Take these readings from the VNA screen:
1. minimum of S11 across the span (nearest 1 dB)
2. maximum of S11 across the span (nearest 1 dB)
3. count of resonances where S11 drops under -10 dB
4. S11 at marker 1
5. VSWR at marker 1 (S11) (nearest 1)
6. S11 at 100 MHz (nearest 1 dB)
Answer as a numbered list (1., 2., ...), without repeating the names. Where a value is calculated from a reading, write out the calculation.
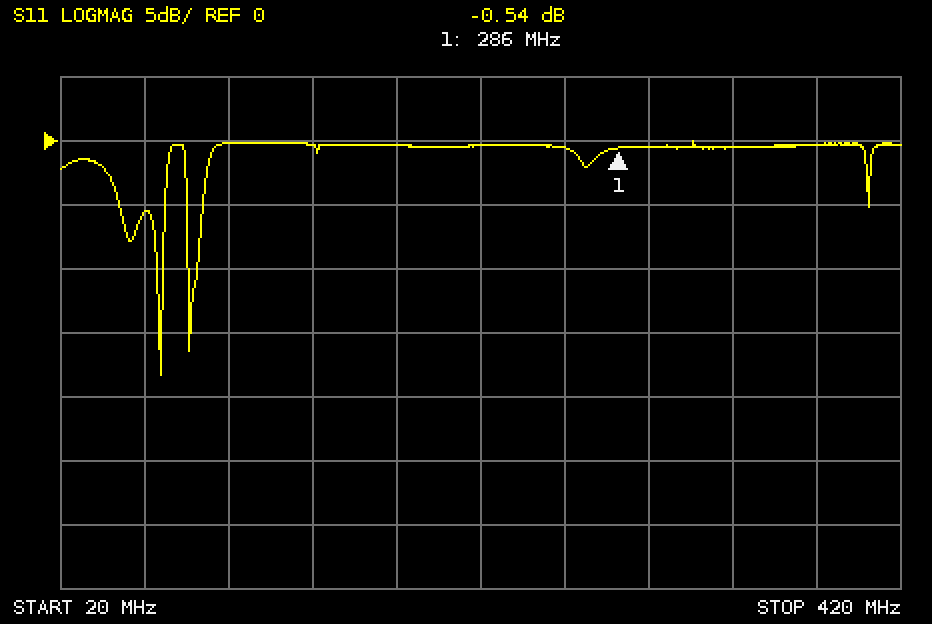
1. -18 dB
2. 0 dB
3. 2
4. -0.54 dB
5. (1 + 0.9397)/(1 − 0.9397) ≈ 32
6. 0 dB
